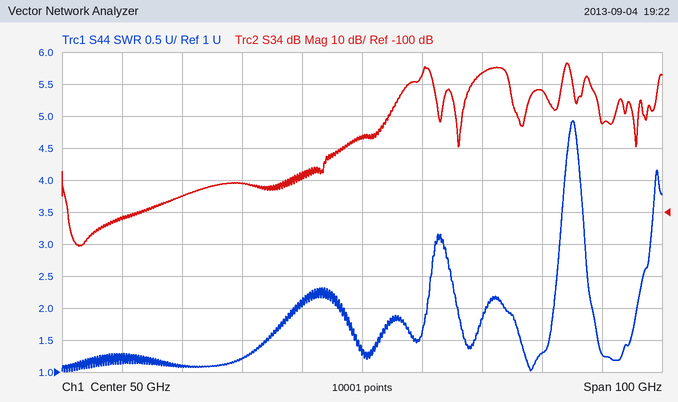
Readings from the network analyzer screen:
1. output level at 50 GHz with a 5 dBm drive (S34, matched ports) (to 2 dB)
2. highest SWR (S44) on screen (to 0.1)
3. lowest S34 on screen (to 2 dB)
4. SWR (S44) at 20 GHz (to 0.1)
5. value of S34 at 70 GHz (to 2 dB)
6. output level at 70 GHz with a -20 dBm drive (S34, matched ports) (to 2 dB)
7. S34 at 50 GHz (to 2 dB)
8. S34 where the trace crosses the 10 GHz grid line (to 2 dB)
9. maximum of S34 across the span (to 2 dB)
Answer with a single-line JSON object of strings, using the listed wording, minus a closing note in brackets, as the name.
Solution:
{"output level at 50 GHz with a 5 dBm drive (S34, matched ports)": "-72 dBm", "highest SWR (S44) on screen": "4.9", "lowest S34 on screen": "-110 dB", "SWR (S44) at 20 GHz": "1.1", "value of S34 at 70 GHz": "-56 dB", "output level at 70 GHz with a -20 dBm drive (S34, matched ports)": "-76 dBm", "S34 at 50 GHz": "-76 dB", "S34 where the trace crosses the 10 GHz grid line": "-102 dB", "maximum of S34 across the span": "-54 dB"}
